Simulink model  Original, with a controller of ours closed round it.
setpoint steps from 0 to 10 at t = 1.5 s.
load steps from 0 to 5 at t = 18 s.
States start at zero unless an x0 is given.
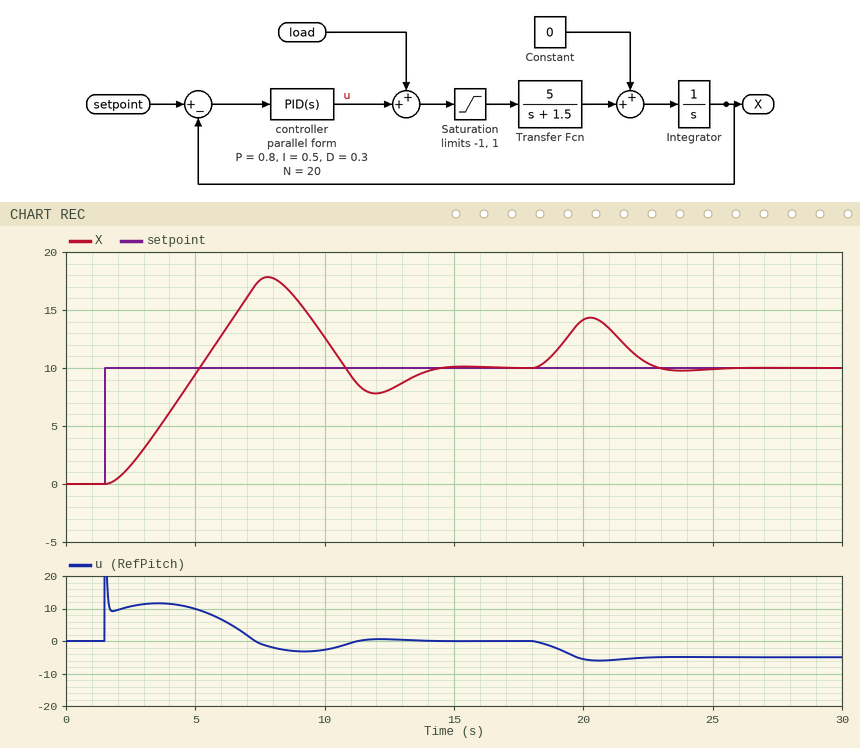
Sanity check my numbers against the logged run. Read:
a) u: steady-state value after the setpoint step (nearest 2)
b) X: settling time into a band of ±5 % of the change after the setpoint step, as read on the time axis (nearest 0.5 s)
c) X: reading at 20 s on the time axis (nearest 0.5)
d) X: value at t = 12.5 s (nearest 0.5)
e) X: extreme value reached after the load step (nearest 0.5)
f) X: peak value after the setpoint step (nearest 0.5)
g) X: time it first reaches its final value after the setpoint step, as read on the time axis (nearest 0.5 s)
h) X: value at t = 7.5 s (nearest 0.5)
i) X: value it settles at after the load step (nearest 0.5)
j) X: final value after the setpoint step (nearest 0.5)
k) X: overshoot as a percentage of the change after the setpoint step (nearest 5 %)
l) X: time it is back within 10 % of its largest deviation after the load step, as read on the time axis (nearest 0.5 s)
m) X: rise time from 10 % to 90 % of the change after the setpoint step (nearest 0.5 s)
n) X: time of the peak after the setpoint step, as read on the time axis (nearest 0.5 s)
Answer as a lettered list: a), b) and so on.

a) 0
b) 13.5 s
c) 14.0
d) 8.0
e) 14.5
f) 18.0
g) 5.0 s
h) 17.5
i) 10.0
j) 10.0
k) 80 %
l) 22.5 s
m) 2.5 s
n) 8.0 s
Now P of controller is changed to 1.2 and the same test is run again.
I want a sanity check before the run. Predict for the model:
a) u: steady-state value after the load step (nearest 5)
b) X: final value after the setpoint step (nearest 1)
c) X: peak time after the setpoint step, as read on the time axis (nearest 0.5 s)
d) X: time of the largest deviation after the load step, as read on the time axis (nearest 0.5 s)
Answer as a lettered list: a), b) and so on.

a) -5
b) 10
c) 7.5 s
d) 20.0 s
